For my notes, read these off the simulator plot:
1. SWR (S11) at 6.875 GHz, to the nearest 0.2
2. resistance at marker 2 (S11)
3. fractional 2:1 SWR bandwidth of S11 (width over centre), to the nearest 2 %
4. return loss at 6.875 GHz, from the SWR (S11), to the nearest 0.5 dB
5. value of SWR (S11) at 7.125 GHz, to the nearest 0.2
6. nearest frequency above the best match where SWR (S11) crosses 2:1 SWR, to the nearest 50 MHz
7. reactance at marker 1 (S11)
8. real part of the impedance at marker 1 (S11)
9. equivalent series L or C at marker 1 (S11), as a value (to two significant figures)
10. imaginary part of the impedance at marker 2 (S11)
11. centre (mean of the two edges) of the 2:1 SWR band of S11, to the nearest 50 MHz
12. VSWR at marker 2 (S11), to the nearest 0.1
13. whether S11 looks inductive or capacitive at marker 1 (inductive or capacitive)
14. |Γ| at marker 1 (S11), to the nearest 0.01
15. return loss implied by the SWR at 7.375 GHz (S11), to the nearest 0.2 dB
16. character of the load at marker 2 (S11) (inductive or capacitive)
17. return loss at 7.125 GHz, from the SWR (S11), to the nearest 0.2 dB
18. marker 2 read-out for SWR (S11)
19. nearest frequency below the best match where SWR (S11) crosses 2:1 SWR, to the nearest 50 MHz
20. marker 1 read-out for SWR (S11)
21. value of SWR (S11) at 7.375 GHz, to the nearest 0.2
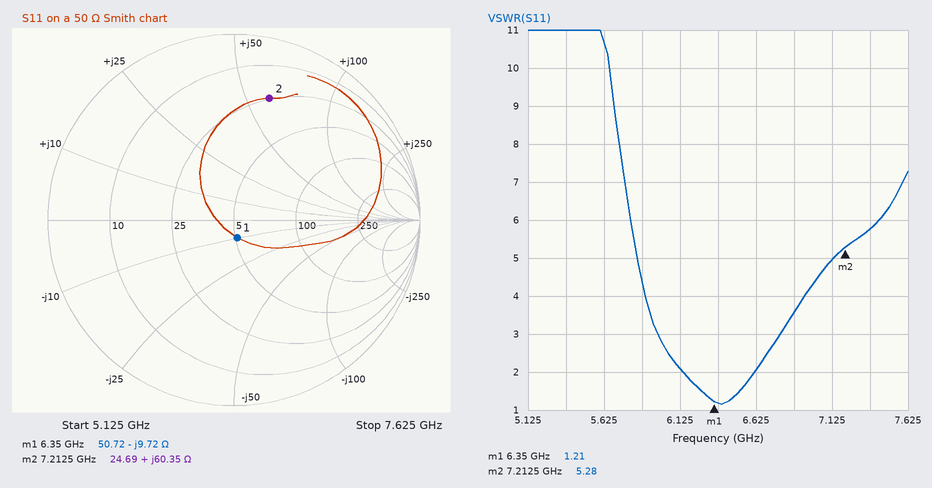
3.6
24.69 Ω
8 %
5.0 dB
5.0
6.60 GHz
-9.72 Ω
50.72 Ω
2.6 pF
+60.35 Ω
6.40 GHz
5.3
capacitive
0.10
3.0 dB
inductive
3.6 dB
5.28
6.15 GHz
1.21
5.8
